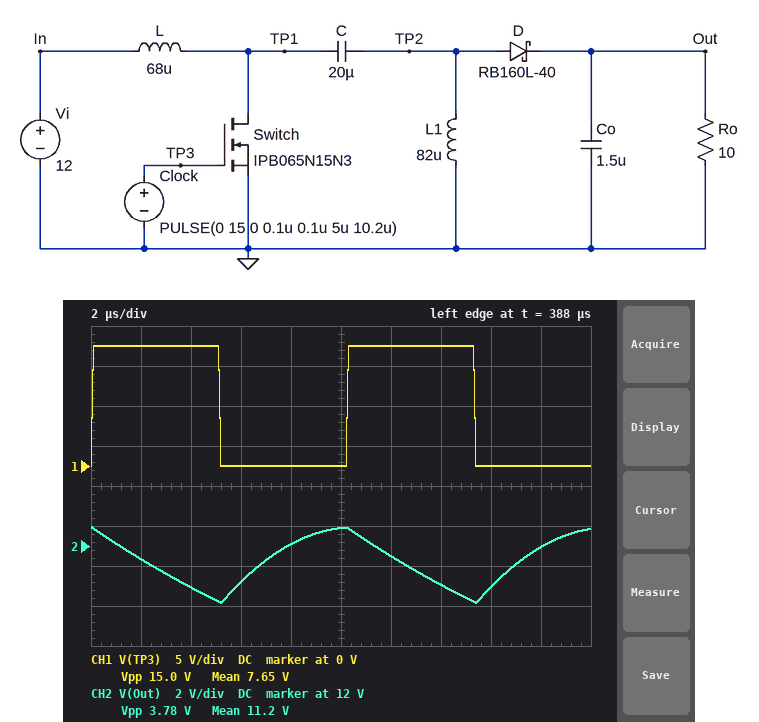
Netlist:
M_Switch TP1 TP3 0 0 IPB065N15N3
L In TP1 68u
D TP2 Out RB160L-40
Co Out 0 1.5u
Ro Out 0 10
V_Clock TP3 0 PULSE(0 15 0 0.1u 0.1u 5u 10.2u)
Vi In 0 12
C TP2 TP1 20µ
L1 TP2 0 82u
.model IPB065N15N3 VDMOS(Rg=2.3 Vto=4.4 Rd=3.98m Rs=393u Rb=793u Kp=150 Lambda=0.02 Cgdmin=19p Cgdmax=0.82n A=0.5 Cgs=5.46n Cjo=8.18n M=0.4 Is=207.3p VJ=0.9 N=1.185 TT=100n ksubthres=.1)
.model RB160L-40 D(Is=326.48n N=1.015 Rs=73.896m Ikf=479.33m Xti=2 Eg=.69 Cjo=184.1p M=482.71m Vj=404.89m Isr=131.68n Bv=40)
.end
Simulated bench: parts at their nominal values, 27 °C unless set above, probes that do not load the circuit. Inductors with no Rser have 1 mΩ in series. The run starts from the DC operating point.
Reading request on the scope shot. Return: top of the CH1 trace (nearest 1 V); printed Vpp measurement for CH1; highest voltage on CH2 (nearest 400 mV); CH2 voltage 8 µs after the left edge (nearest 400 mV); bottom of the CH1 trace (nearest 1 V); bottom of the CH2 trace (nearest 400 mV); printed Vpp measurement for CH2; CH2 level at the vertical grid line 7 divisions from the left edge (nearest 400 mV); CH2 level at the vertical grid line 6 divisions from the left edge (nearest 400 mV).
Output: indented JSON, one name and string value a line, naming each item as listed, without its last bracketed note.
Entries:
{
  "top of the CH1 trace": "15 V",
  "printed Vpp measurement for CH1": "15.0 V",
  "highest voltage on CH2": "12.8 V",
  "CH2 voltage 8 µs after the left edge": "12.0 V",
  "bottom of the CH1 trace": "0 V",
  "bottom of the CH2 trace": "9.2 V",
  "printed Vpp measurement for CH2": "3.78 V",
  "CH2 level at the vertical grid line 7 divisions from the left edge": "10.0 V",
  "CH2 level at the vertical grid line 6 divisions from the left edge": "11.6 V"
}
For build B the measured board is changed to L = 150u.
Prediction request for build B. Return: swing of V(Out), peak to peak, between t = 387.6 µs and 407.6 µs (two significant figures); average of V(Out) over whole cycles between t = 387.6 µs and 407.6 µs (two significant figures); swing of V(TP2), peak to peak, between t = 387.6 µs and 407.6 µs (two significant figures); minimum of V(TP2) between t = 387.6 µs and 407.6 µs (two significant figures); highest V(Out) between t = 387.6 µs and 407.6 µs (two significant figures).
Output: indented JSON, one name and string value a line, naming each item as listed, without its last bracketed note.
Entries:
{
  "swing of V(Out), peak to peak, between t = 387.6 µs and 407.6 µs": "3.9 V",
  "average of V(Out) over whole cycles between t = 387.6 µs and 407.6 µs": "12 V",
  "swing of V(TP2), peak to peak, between t = 387.6 µs and 407.6 µs": "27 V",
  "minimum of V(TP2) between t = 387.6 µs and 407.6 µs": "-13 V",
  "highest V(Out) between t = 387.6 µs and 407.6 µs": "13 V"
}
